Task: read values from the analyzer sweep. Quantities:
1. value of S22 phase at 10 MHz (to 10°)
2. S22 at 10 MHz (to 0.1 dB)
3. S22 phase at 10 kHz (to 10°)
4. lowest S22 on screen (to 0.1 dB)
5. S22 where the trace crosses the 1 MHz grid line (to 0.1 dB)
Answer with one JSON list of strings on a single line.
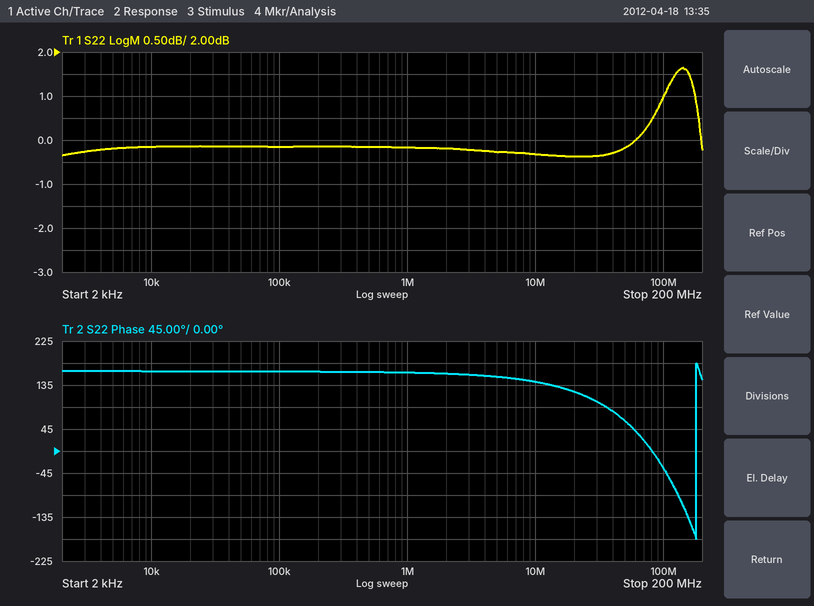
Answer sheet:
["140°", "-0.3 dB", "160°", "-0.4 dB", "-0.2 dB"]
